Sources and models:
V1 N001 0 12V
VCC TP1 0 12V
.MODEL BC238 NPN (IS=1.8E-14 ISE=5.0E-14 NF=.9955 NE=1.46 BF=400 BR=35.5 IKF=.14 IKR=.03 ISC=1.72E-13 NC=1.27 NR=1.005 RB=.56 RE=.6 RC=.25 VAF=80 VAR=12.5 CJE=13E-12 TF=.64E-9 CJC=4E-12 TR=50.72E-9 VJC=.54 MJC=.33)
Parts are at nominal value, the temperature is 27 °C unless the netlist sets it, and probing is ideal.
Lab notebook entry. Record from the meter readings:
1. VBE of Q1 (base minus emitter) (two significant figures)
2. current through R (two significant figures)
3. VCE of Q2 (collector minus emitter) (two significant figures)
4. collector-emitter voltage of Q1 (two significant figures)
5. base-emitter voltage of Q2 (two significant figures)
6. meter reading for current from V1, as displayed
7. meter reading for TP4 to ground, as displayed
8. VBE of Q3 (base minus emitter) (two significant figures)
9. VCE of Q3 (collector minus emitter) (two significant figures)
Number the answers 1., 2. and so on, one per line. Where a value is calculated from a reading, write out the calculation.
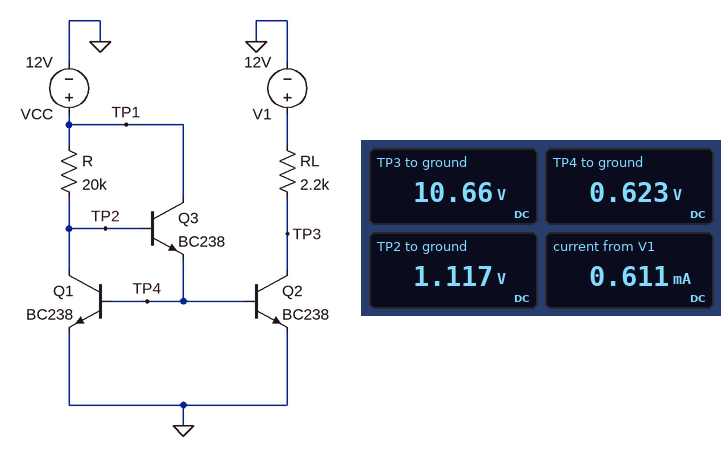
1. 623 mV = 620 mV
2. (12 V - 1.117 V) / 20 kΩ = 540 µA
3. 10.66 V = 11 V
4. 1.117 V = 1.1 V
5. 623 mV = 620 mV
6. 0.611 mA
7. 0.623 V
8. 1.117 V - 623 mV = 490 mV
9. 12 V - 623 mV = 11 V
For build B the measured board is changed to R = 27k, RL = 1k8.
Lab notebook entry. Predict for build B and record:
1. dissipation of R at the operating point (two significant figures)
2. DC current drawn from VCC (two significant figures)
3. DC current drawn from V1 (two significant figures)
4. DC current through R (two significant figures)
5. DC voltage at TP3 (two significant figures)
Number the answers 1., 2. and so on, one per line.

1. 4.4 mW
2. 410 µA
3. 460 µA
4. 400 µA
5. 11 V
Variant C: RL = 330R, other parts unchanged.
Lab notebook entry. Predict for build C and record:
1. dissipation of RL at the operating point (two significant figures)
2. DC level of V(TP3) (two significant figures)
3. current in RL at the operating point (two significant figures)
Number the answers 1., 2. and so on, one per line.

1. 130 µW
2. 12 V
3. 620 µA
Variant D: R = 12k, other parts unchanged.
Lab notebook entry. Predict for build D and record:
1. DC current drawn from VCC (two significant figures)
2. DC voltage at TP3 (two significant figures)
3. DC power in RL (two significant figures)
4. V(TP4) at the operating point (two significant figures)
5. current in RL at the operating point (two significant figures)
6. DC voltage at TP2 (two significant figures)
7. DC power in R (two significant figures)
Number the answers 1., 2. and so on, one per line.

1. 910 µA
2. 9.8 V
3. 2.2 mW
4. 640 mV
5. 1.0 mA
6. 1.1 V
7. 9.8 mW
